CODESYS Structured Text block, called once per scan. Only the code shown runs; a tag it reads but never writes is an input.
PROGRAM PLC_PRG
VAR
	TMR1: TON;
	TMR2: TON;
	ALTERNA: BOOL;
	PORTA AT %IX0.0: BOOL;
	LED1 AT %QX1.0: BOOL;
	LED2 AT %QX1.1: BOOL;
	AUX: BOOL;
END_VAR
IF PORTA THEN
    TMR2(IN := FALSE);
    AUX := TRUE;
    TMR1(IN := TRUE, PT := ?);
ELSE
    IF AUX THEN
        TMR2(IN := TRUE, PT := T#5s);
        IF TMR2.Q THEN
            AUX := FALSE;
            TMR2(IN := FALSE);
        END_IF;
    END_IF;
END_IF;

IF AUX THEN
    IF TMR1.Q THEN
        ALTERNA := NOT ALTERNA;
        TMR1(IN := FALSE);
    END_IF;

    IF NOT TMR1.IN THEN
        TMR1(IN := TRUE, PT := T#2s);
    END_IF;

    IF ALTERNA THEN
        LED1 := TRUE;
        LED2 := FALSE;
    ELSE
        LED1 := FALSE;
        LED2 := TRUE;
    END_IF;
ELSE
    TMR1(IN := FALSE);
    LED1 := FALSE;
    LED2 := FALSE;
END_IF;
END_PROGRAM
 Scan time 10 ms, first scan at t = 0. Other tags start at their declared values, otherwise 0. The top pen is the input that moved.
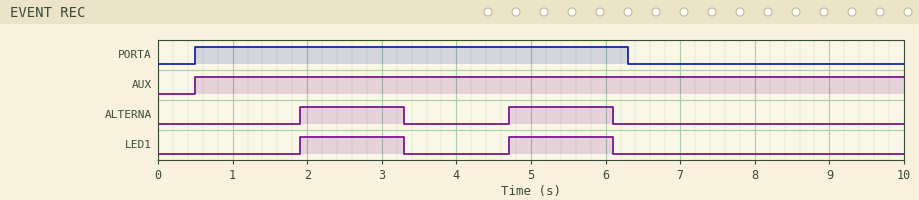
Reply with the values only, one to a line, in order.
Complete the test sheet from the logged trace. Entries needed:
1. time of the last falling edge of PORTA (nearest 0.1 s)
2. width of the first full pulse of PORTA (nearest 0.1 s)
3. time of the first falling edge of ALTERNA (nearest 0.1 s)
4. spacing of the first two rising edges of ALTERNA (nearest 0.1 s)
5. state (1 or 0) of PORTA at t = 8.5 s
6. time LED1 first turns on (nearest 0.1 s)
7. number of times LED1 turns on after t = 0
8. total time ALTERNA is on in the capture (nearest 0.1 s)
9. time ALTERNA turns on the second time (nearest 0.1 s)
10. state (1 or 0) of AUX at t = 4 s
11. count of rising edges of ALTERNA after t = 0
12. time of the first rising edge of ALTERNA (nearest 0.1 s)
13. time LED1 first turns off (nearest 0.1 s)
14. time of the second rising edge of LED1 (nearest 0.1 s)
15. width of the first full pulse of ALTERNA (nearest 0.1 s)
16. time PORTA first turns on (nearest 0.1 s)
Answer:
6.3 s
5.8 s
3.3 s
2.8 s
0
1.9 s
2
2.8 s
4.7 s
1
2
1.9 s
3.3 s
4.7 s
1.4 s
0.5 s
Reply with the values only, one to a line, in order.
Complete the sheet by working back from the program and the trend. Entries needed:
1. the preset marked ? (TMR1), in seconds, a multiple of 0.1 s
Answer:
1.4 s
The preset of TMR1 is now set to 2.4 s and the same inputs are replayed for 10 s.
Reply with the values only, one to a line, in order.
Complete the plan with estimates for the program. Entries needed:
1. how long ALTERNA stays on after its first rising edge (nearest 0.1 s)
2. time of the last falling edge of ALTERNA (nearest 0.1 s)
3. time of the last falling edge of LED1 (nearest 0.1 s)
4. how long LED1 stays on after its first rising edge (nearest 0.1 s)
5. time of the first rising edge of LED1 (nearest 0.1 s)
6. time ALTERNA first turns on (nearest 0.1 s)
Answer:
2.4 s
5.3 s
5.3 s
2.4 s
2.9 s
2.9 s
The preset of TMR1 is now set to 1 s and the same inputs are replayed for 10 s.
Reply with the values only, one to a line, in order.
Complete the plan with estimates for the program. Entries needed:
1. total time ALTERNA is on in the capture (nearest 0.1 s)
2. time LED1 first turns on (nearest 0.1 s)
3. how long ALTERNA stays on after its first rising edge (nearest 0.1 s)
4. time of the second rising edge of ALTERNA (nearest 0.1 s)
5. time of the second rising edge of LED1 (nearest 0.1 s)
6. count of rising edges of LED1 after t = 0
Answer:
6.5 s
1.5 s
1.0 s
3.5 s
3.5 s
3
